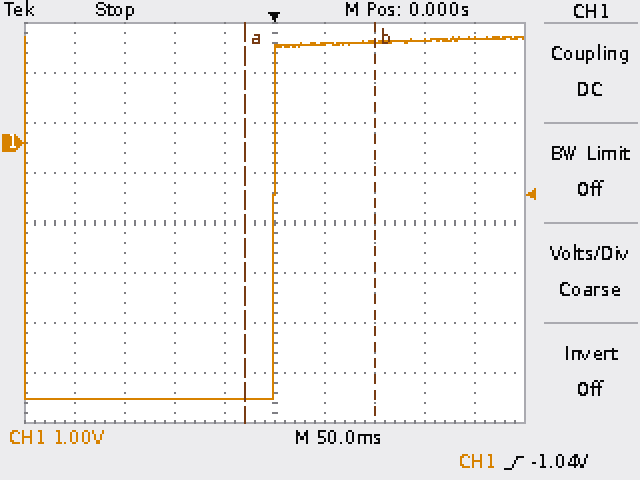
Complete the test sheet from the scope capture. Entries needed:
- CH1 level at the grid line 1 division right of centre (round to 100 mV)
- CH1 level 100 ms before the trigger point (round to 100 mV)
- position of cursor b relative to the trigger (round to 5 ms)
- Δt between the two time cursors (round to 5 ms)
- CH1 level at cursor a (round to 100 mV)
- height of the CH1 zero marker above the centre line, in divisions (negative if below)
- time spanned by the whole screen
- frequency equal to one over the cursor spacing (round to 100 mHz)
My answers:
2.0 V
-5.1 V
+100 ms
130 ms
-5.1 V
+1.6 div
500 ms
7.7 Hz
